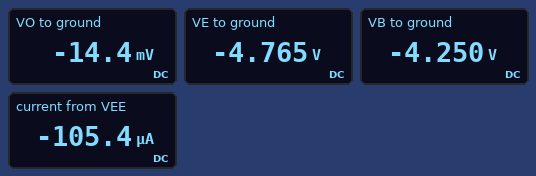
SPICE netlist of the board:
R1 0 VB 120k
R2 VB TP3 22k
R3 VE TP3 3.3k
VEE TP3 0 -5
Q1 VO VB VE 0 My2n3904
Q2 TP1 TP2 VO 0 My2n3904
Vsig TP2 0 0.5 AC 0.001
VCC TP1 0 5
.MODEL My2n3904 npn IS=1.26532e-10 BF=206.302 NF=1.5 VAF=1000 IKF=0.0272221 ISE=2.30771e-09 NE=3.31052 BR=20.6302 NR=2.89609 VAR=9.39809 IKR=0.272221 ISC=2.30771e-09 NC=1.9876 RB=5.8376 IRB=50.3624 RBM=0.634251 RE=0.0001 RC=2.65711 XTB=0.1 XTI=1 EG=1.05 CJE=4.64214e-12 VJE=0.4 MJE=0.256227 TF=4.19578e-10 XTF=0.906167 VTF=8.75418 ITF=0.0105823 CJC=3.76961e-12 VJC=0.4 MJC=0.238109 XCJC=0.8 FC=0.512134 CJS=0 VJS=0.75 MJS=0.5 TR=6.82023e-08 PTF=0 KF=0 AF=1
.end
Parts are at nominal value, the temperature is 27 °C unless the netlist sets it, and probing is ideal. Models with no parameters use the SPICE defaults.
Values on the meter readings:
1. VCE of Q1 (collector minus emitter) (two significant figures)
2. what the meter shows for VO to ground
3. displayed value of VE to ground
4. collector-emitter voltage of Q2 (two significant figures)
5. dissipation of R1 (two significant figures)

4.8 V
-14.4 mV
-4.765 V
5.0 V
150 µW
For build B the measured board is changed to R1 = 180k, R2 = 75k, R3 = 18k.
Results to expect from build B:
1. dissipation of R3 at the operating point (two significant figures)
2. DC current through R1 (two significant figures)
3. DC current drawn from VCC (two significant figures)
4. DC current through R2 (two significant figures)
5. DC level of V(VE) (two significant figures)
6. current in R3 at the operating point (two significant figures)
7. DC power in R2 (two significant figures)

46 µW
20 µA
49 µA
19 µA
-4.1 V
51 µA
27 µW
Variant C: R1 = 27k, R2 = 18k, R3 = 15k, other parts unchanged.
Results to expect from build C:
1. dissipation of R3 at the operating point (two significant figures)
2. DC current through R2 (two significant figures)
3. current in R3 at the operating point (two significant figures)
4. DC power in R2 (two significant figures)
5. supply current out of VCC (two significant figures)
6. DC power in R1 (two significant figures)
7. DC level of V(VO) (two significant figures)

140 µW
110 µA
97 µA
220 µW
94 µA
340 µW
-27 mV
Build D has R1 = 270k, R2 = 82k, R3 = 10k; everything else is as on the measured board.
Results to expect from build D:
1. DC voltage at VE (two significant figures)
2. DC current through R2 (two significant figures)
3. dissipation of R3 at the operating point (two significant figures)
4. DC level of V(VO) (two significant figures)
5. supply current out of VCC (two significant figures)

-4.4 V
13 µA
34 µW
-6.6 mV
56 µA
